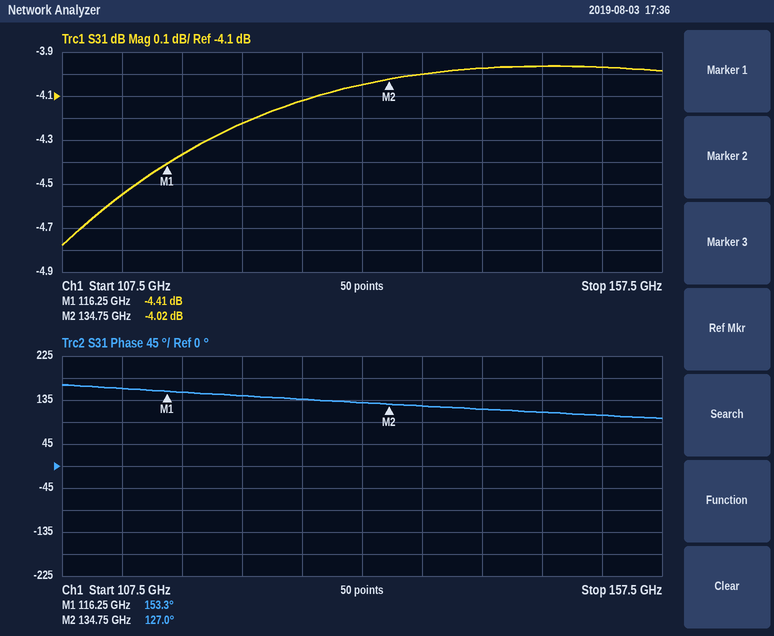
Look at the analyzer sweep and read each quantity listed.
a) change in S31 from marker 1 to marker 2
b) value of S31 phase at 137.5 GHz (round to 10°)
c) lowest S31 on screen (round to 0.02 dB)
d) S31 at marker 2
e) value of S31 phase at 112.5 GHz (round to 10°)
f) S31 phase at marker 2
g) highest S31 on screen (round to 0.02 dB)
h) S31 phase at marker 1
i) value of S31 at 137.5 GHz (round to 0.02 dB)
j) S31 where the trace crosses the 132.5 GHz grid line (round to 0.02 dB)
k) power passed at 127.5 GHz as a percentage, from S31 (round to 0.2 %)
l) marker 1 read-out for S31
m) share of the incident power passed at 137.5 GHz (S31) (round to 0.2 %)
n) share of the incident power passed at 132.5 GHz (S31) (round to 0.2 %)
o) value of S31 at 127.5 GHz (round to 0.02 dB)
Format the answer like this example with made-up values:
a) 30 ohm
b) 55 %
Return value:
a) 0.39 dB
b) 120°
c) -4.78 dB
d) -4.02 dB
e) 160°
f) 127.0°
g) -3.96 dB
h) 153.3°
i) -4.00 dB
j) -4.04 dB
k) 38.8 %
l) -4.41 dB
m) 39.8 %
n) 39.4 %
o) -4.12 dB
